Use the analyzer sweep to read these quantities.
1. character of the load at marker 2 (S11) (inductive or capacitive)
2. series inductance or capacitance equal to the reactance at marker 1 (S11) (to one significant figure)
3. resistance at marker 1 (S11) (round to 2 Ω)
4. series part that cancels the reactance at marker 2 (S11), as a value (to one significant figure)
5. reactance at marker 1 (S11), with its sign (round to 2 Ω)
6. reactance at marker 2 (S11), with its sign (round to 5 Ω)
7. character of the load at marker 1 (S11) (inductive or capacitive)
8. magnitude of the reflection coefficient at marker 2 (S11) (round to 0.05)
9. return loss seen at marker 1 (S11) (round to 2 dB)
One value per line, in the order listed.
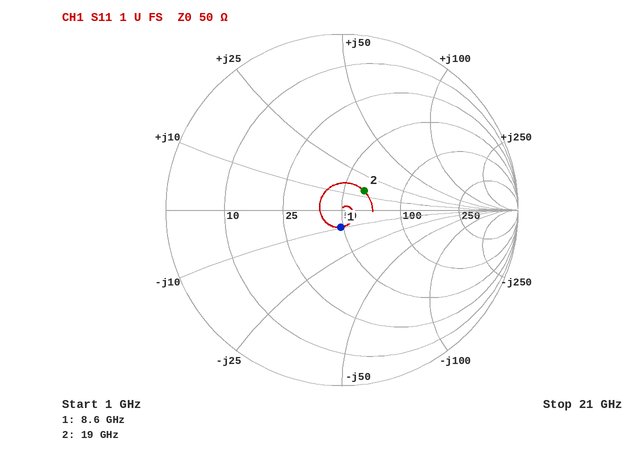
inductive
2 pF
48 Ω
600 fF
-10 Ω
+15 Ω
capacitive
0.15
20 dB
